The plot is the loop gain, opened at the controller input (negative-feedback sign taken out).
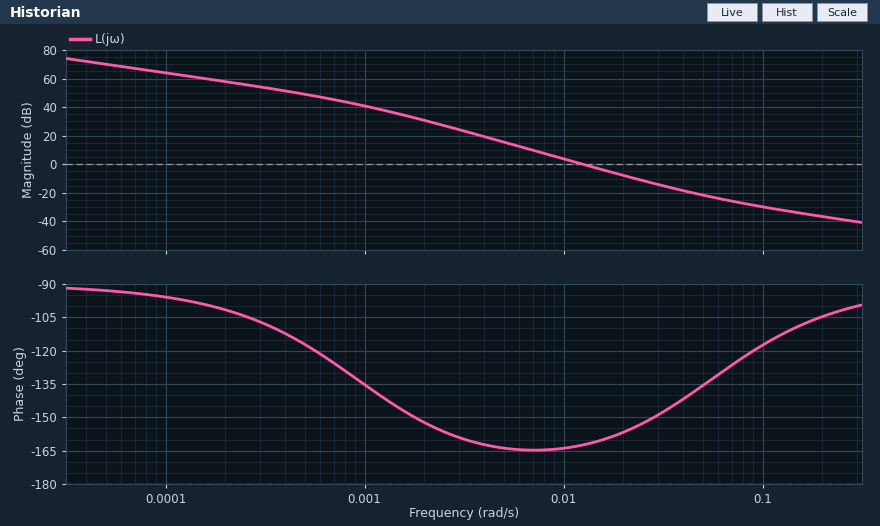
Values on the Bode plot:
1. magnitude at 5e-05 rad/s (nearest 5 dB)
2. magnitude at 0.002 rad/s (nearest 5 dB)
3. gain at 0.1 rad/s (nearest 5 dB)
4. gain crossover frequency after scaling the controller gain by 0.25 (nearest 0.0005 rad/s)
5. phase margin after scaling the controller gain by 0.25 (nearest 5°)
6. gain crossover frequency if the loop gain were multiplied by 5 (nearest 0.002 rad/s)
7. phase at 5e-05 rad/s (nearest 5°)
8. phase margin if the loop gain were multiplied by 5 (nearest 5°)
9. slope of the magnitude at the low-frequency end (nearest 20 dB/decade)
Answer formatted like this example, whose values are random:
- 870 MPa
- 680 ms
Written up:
- 70 dB
- 30 dB
- -30 dB
- 0.0060 rad/s
- 15°
- 0.030 rad/s
- -95°
- 30°
- -20 dB/decade
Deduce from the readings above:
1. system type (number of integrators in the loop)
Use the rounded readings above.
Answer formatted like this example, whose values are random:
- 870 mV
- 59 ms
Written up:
- 1
